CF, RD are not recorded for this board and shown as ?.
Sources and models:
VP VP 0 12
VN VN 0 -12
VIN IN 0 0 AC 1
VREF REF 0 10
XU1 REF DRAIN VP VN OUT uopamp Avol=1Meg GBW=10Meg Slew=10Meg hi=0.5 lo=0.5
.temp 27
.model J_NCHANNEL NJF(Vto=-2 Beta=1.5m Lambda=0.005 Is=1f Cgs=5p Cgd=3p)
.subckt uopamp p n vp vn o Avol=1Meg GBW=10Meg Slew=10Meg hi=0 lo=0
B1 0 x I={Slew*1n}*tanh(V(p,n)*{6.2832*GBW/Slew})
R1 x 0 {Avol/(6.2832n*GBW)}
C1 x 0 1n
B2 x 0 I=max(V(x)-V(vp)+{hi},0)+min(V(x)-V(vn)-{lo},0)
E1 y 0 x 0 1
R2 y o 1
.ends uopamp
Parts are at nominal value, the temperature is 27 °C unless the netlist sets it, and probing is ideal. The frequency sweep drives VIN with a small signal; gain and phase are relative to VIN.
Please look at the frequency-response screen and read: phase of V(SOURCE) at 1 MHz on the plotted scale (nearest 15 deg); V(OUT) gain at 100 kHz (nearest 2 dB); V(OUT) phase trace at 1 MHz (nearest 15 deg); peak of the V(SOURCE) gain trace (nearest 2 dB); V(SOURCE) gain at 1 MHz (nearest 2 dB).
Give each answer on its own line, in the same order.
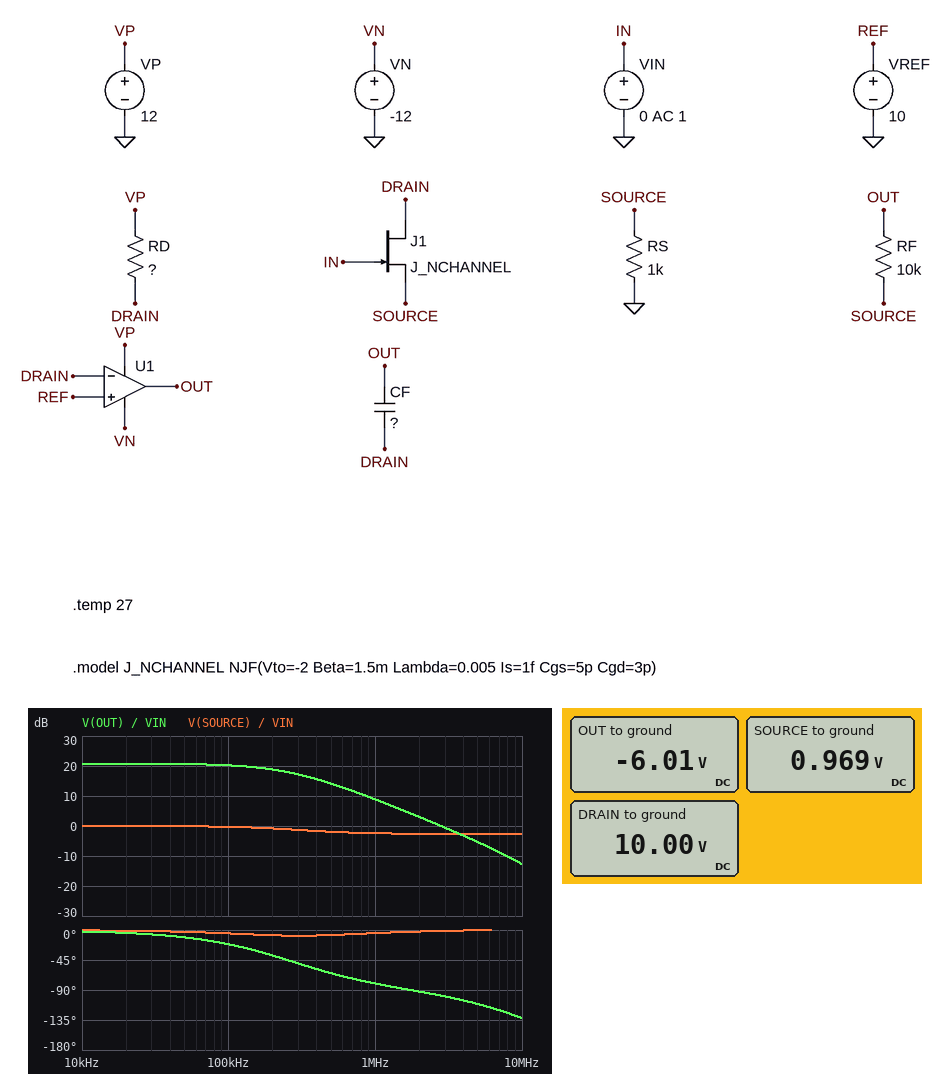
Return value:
0 deg
20 dB
-75 deg
0 dB
-2 dB
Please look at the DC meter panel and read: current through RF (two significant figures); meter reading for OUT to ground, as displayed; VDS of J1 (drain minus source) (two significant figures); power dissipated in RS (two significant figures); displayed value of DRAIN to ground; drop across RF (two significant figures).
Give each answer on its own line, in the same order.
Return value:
700 µA
-6.01 V
9.0 V
940 µW
10.00 V
7.0 V
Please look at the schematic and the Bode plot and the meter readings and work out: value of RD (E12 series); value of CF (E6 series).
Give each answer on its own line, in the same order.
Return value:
1.2 kΩ
33 pF
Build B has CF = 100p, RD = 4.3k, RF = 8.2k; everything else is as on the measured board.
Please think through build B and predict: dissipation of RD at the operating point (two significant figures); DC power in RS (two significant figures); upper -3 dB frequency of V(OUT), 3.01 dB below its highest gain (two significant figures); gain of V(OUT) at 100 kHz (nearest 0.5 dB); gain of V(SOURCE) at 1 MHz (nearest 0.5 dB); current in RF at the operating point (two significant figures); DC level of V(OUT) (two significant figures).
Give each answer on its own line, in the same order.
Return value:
930 µW
2.1 mW
110 kHz
17.0 dB
-4.5 dB
990 µA
9.6 V
